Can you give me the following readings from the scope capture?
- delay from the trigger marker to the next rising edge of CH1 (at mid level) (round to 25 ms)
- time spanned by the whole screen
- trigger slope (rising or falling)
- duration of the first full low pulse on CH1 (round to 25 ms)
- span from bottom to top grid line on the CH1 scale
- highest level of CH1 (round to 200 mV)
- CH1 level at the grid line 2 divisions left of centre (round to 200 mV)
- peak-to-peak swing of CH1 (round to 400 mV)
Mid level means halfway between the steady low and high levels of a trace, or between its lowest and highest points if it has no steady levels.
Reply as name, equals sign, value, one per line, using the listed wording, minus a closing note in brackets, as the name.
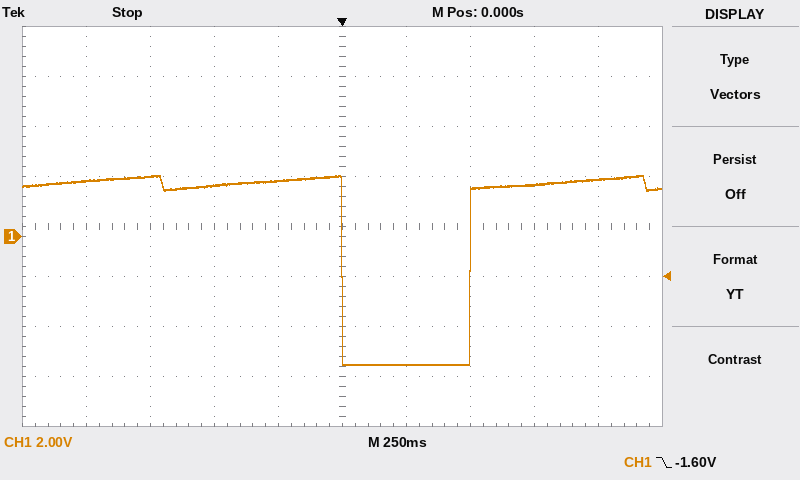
delay from the trigger marker to the next rising edge of CH1 (at mid level) = 500 ms
time spanned by the whole screen = 2.5 s
trigger slope = falling
duration of the first full low pulse on CH1 = 500 ms
span from bottom to top grid line on the CH1 scale = 16 V
highest level of CH1 = 2.4 V
CH1 level at the grid line 2 divisions left of centre = 2.0 V
peak-to-peak swing of CH1 = 7.6 V
